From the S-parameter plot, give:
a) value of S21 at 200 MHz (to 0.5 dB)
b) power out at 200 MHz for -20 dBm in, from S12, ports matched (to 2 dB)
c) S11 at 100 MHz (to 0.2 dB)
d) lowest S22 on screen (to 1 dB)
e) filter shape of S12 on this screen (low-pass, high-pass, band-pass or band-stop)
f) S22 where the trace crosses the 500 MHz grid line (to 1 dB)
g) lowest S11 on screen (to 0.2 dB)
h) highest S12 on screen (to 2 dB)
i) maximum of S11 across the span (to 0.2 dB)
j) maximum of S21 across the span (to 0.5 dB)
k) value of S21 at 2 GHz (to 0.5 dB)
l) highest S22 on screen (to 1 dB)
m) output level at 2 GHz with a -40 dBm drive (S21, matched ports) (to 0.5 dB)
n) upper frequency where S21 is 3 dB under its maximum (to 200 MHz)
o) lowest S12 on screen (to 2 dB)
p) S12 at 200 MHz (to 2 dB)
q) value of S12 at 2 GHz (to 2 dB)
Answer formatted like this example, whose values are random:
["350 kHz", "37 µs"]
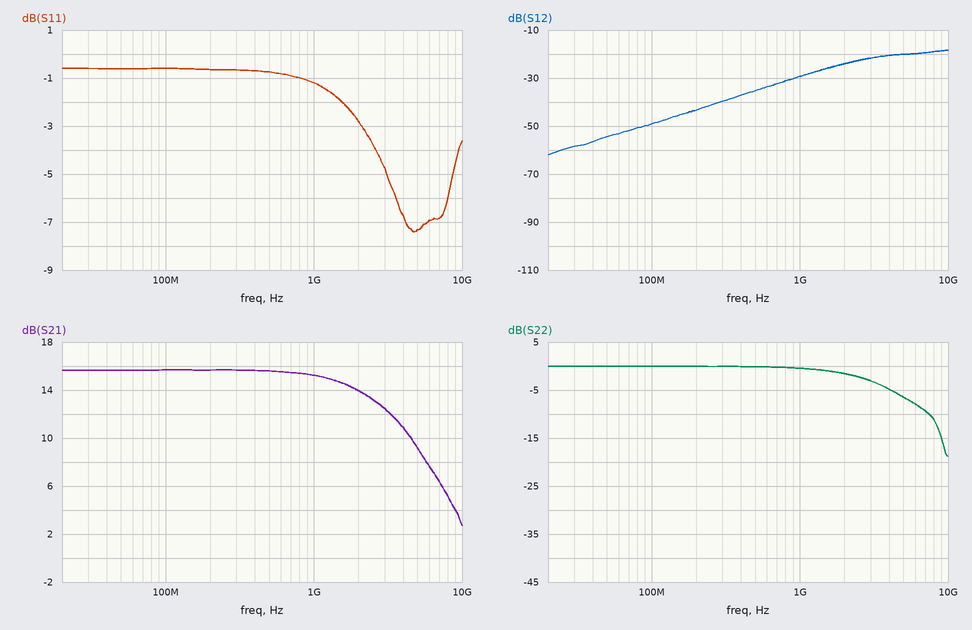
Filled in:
["15.5 dB", "-64 dBm", "-0.6 dB", "-19 dB", "high-pass", "0 dB", "-7.4 dB", "-18 dB", "-0.6 dB", "15.5 dB", "14.0 dB", "0 dB", "-26.0 dBm", "2.8 GHz", "-62 dB", "-44 dB", "-24 dB"]
